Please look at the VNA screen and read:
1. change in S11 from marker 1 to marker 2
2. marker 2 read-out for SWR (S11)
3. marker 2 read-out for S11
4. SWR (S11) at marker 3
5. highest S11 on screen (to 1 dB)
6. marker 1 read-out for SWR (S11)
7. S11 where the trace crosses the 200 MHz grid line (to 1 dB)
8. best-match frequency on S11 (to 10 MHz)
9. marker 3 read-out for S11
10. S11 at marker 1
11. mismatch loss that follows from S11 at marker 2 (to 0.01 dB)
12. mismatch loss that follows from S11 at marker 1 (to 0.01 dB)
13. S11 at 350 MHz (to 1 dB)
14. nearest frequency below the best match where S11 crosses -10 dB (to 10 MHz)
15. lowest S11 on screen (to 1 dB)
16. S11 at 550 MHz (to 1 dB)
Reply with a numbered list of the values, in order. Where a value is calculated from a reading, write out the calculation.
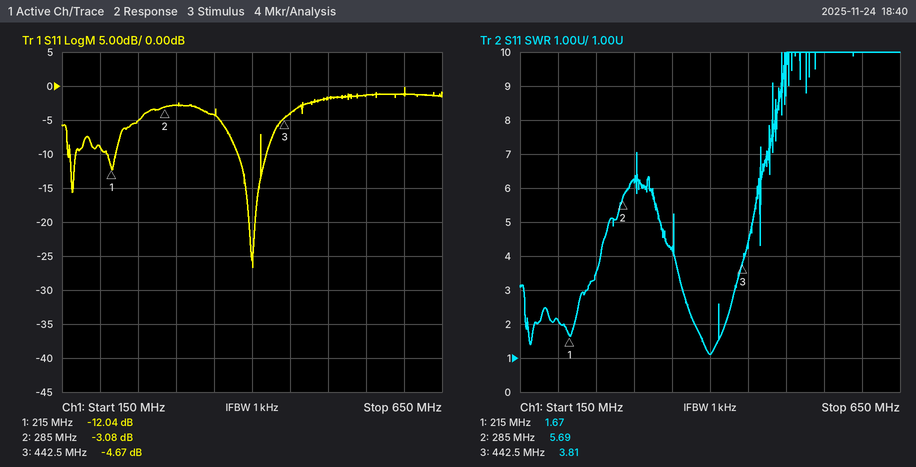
1. -3.08 − (-12.04) = 8.96 dB
2. 5.69
3. -3.08 dB
4. 3.81
5. 0 dB
6. 1.67
7. -9 dB
8. 400 MHz
9. -4.67 dB
10. -12.04 dB
11. −10 log10(1 − 10^(-3.08/10)) ≈ 2.94 dB
12. −10 log10(1 − 10^(-12.04/10)) ≈ 0.28 dB
13. -4 dB
14. 380 MHz
15. -27 dB
16. -1 dB
